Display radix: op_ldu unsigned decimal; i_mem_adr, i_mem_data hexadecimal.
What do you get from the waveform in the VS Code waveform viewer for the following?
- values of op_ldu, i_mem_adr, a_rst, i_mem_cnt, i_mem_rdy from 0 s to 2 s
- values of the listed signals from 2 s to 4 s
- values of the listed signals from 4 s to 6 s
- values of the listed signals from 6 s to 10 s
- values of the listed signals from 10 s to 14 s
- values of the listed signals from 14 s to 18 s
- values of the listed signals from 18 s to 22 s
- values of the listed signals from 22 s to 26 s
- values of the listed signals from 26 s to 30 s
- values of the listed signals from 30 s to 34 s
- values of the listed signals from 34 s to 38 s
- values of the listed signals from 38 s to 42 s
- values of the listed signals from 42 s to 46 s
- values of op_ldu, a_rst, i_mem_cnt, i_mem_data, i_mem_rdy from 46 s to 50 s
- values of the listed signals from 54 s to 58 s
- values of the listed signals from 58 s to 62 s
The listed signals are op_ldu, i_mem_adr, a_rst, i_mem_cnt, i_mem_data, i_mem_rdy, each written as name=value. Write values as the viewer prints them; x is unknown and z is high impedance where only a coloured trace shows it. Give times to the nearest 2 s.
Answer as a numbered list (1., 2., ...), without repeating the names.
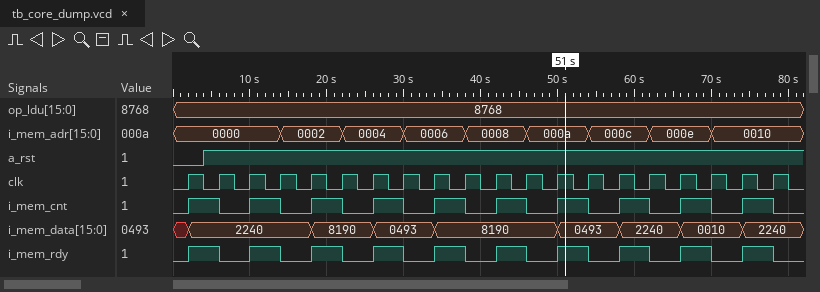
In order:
1. op_ldu=8768, i_mem_adr=0000, a_rst=0, i_mem_cnt=0, i_mem_rdy=0
2. op_ldu=8768, i_mem_adr=0000, a_rst=0, i_mem_cnt=1, i_mem_data=2240, i_mem_rdy=1
3. op_ldu=8768, i_mem_adr=0000, a_rst=1, i_mem_cnt=1, i_mem_data=2240, i_mem_rdy=1
4. op_ldu=8768, i_mem_adr=0000, a_rst=1, i_mem_cnt=0, i_mem_data=2240, i_mem_rdy=0
5. op_ldu=8768, i_mem_adr=0000, a_rst=1, i_mem_cnt=1, i_mem_data=2240, i_mem_rdy=1
6. op_ldu=8768, i_mem_adr=0002, a_rst=1, i_mem_cnt=0, i_mem_data=2240, i_mem_rdy=0
7. op_ldu=8768, i_mem_adr=0002, a_rst=1, i_mem_cnt=1, i_mem_data=8190, i_mem_rdy=1
8. op_ldu=8768, i_mem_adr=0004, a_rst=1, i_mem_cnt=0, i_mem_data=8190, i_mem_rdy=0
9. op_ldu=8768, i_mem_adr=0004, a_rst=1, i_mem_cnt=1, i_mem_data=0493, i_mem_rdy=1
10. op_ldu=8768, i_mem_adr=0006, a_rst=1, i_mem_cnt=0, i_mem_data=0493, i_mem_rdy=0
11. op_ldu=8768, i_mem_adr=0006, a_rst=1, i_mem_cnt=1, i_mem_data=8190, i_mem_rdy=1
12. op_ldu=8768, i_mem_adr=0008, a_rst=1, i_mem_cnt=0, i_mem_data=8190, i_mem_rdy=0
13. op_ldu=8768, i_mem_adr=0008, a_rst=1, i_mem_cnt=1, i_mem_data=8190, i_mem_rdy=1
14. op_ldu=8768, a_rst=1, i_mem_cnt=0, i_mem_data=8190, i_mem_rdy=0
15. op_ldu=8768, i_mem_adr=000c, a_rst=1, i_mem_cnt=0, i_mem_data=0493, i_mem_rdy=0
16. op_ldu=8768, i_mem_adr=000c, a_rst=1, i_mem_cnt=1, i_mem_data=2240, i_mem_rdy=1
